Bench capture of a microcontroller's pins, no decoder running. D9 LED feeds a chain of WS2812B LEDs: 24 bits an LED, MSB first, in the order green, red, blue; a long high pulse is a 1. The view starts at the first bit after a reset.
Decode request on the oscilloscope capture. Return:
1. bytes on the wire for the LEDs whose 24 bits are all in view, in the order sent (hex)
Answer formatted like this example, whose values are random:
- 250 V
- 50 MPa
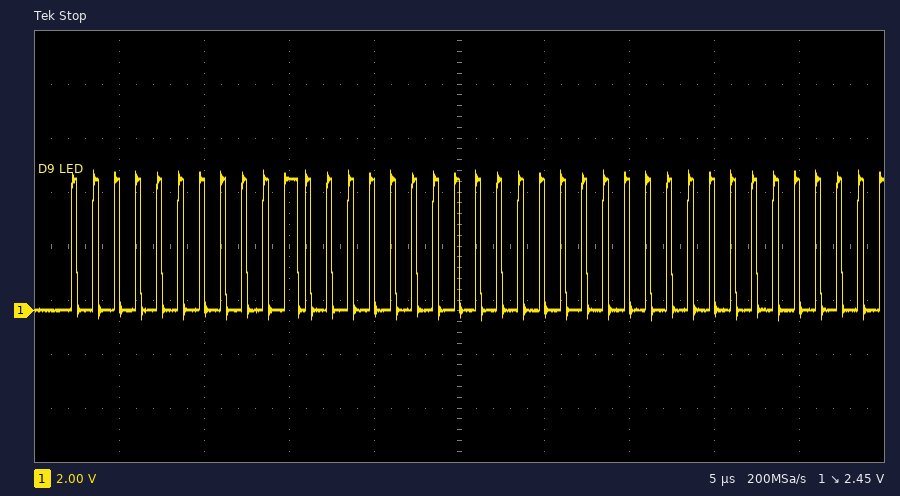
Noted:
- 00 20 00
